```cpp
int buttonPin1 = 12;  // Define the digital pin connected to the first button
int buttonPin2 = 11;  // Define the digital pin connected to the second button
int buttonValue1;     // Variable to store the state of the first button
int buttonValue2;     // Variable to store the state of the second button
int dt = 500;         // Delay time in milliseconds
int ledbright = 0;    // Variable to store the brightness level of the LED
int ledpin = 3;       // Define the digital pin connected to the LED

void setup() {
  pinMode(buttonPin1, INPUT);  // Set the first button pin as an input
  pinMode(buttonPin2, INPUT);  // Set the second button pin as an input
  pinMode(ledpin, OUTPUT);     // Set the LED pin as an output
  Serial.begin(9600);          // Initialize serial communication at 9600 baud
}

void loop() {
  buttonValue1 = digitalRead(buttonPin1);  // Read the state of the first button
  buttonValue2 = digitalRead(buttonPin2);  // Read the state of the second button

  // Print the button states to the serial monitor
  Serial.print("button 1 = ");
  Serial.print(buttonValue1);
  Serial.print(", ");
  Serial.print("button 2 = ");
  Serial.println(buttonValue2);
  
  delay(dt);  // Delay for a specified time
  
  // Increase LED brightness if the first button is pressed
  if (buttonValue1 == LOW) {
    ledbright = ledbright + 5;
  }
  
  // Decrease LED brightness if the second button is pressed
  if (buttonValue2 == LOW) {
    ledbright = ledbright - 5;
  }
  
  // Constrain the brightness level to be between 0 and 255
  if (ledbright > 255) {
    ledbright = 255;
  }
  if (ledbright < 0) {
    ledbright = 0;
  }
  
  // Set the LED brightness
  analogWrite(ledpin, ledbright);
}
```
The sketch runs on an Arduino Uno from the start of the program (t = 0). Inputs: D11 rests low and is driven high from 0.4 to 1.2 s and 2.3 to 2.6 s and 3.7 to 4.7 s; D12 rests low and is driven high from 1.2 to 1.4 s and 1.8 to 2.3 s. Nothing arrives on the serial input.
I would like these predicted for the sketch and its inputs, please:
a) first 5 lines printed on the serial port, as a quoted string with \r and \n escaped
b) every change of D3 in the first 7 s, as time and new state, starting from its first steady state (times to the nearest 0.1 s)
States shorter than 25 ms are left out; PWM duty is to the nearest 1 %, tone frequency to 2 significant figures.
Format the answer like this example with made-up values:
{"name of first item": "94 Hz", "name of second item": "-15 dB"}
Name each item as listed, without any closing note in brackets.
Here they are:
{"first 5 lines printed on the serial port, as a quoted string with \\r and \\n escaped": "\"button 1 = 0, button 2 = 0\\r\\nbutton 1 = 0, button 2 = 1\\r\\nbutton 1 = 0, button 2 = 1\\r\\nbutton 1 = 0, button 2 = 0\\r\\nbutton 1 = 1, button 2 = 0\\r\\n\"", "every change of D3 in the first 7 s, as time and new state, starting from its first steady state": "0 s low; 1 s PWM 2 %; 1.5 s PWM 4 %; 2.5 s PWM 2 %; 3 s PWM 4 %; 4.5 s PWM 6 %; 5 s PWM 8 %"}
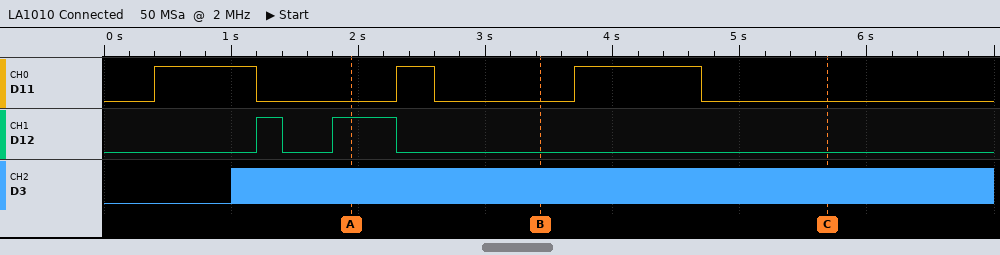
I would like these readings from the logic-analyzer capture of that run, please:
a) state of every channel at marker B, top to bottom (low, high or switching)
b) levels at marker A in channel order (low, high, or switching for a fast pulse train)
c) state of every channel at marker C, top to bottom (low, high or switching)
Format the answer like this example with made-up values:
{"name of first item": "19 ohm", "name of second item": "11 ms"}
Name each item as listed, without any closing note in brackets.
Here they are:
{"state of every channel at marker B, top to bottom": "D11 low, D12 low, D3 switching", "levels at marker A in channel order": "D11 low, D12 high, D3 switching", "state of every channel at marker C, top to bottom": "D11 low, D12 low, D3 switching"}
